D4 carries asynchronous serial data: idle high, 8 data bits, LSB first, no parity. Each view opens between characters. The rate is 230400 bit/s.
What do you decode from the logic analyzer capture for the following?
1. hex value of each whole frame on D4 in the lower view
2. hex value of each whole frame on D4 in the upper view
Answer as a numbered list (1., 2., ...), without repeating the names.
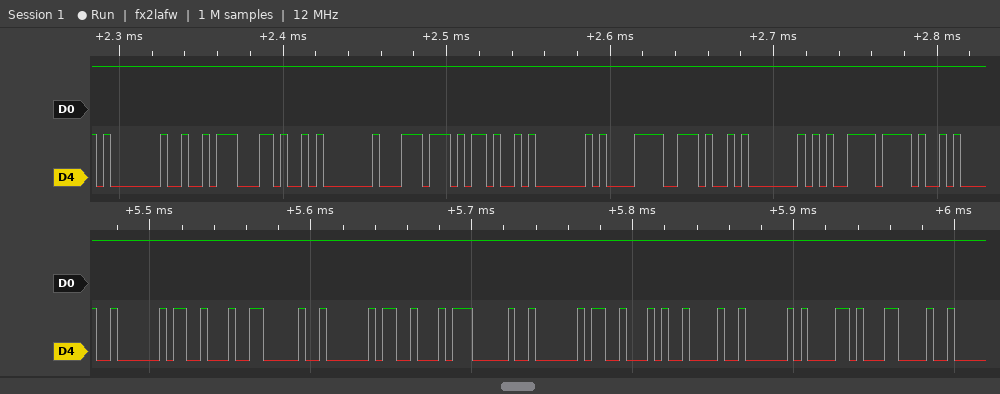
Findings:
1. 02, 13, 06, 02, 13, 07, 02, 13, 09, 02, 61, 0C
2. 01, D2, 2C, 01, DC, 2D, 01, E1, 2E, 01, E5, 2F
